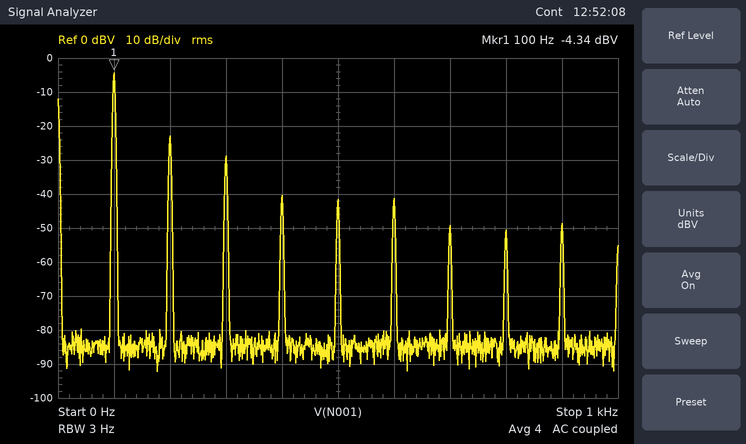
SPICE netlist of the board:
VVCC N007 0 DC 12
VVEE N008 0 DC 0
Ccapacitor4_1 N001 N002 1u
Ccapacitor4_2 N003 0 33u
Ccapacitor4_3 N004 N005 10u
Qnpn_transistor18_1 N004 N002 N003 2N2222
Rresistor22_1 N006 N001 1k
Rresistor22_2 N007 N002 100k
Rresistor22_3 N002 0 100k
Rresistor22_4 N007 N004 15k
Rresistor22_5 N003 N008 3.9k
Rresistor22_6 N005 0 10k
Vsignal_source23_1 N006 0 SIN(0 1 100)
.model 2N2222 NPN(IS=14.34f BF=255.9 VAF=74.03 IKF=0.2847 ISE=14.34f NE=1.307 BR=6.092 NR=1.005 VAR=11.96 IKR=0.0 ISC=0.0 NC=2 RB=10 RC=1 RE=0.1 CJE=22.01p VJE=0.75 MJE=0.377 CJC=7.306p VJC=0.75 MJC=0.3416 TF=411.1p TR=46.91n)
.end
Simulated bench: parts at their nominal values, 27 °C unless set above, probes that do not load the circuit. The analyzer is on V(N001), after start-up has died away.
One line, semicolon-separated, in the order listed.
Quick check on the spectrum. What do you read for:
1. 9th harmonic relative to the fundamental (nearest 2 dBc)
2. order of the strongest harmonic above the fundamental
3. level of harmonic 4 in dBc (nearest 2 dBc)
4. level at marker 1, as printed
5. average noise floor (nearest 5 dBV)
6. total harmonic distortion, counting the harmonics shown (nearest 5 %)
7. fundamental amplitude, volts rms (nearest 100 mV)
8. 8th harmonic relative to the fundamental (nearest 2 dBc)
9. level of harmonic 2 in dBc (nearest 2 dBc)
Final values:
-44 dBc; 2; -36 dBc; -4.34 dBV; -85 dBV; 15 %; 600 mV; -46 dBc; -18 dBc
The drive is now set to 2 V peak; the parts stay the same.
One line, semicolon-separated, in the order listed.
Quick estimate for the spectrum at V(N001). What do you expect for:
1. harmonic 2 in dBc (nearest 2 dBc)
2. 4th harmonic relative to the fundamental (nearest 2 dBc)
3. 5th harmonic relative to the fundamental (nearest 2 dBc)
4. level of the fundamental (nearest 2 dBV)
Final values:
-22 dBc; -32 dBc; -42 dBc; 2 dBV
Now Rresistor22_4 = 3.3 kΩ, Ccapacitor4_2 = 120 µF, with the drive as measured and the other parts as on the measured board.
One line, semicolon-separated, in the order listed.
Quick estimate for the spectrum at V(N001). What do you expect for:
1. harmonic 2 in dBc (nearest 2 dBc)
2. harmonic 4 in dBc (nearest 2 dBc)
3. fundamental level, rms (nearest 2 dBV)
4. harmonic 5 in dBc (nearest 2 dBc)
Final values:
-22 dBc; -32 dBc; -4 dBV; -42 dBc
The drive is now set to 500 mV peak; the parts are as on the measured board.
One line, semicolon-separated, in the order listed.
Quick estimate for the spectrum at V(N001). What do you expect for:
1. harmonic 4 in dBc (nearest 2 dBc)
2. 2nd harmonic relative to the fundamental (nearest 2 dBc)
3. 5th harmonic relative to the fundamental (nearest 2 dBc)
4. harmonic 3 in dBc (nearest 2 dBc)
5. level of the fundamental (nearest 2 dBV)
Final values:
-32 dBc; -16 dBc; -34 dBc; -28 dBc; -10 dBV
